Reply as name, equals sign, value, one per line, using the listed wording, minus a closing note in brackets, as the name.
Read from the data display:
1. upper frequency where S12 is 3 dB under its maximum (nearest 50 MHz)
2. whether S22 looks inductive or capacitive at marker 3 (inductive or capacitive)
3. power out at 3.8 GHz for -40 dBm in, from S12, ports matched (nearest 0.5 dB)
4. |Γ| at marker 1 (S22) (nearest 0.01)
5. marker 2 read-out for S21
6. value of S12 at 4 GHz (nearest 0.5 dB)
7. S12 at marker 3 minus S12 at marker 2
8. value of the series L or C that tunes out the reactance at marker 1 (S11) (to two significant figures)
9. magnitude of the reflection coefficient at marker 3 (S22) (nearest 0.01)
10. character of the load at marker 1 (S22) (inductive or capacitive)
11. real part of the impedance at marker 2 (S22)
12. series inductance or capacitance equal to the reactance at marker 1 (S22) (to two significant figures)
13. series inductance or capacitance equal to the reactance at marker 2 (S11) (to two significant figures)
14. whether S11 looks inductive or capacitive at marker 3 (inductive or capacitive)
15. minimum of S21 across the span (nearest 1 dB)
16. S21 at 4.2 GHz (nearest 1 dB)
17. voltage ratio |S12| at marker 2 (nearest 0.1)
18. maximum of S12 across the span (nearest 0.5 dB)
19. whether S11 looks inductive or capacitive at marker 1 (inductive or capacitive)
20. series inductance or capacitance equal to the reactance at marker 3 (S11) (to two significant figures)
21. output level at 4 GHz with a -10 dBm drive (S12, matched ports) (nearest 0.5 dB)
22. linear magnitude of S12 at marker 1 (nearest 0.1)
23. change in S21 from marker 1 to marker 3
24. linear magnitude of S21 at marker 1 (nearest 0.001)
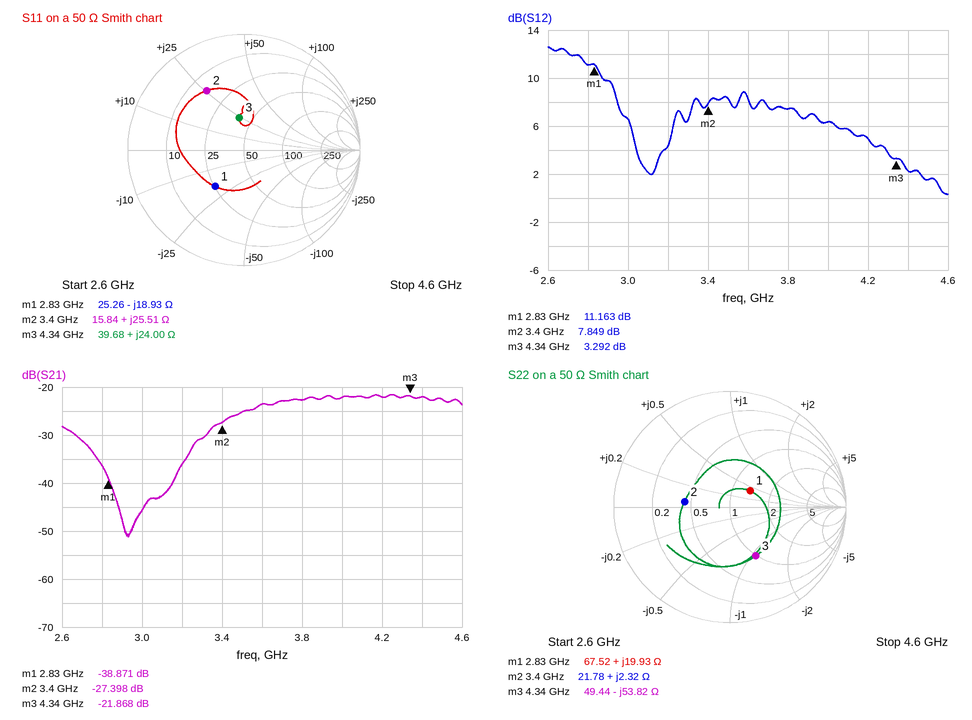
upper frequency where S12 is 3 dB under its maximum = 2.90 GHz
whether S22 looks inductive or capacitive at marker 3 = capacitive
power out at 3.8 GHz for -40 dBm in, from S12, ports matched = -32.5 dBm
|Γ| at marker 1 (S22) = 0.22
marker 2 read-out for S21 = -27.398 dB
value of S12 at 4 GHz = 6.5 dB
S12 at marker 3 minus S12 at marker 2 = -4.557 dB
value of the series L or C that tunes out the reactance at marker 1 (S11) = 1.1 nH
magnitude of the reflection coefficient at marker 3 (S22) = 0.48
character of the load at marker 1 (S22) = inductive
real part of the impedance at marker 2 = 21.78 Ω
series inductance or capacitance equal to the reactance at marker 1 (S22) = 1.1 nH
series inductance or capacitance equal to the reactance at marker 2 (S11) = 1.2 nH
whether S11 looks inductive or capacitive at marker 3 = inductive
minimum of S21 across the span = -51 dB
S21 at 4.2 GHz = -22 dB
voltage ratio |S12| at marker 2 = 2.5
maximum of S12 across the span = 12.5 dB
whether S11 looks inductive or capacitive at marker 1 = capacitive
series inductance or capacitance equal to the reactance at marker 3 (S11) = 880 pH
output level at 4 GHz with a -10 dBm drive (S12, matched ports) = -3.5 dBm
linear magnitude of S12 at marker 1 = 3.6
change in S21 from marker 1 to marker 3 = 17.003 dB
linear magnitude of S21 at marker 1 = 0.011
